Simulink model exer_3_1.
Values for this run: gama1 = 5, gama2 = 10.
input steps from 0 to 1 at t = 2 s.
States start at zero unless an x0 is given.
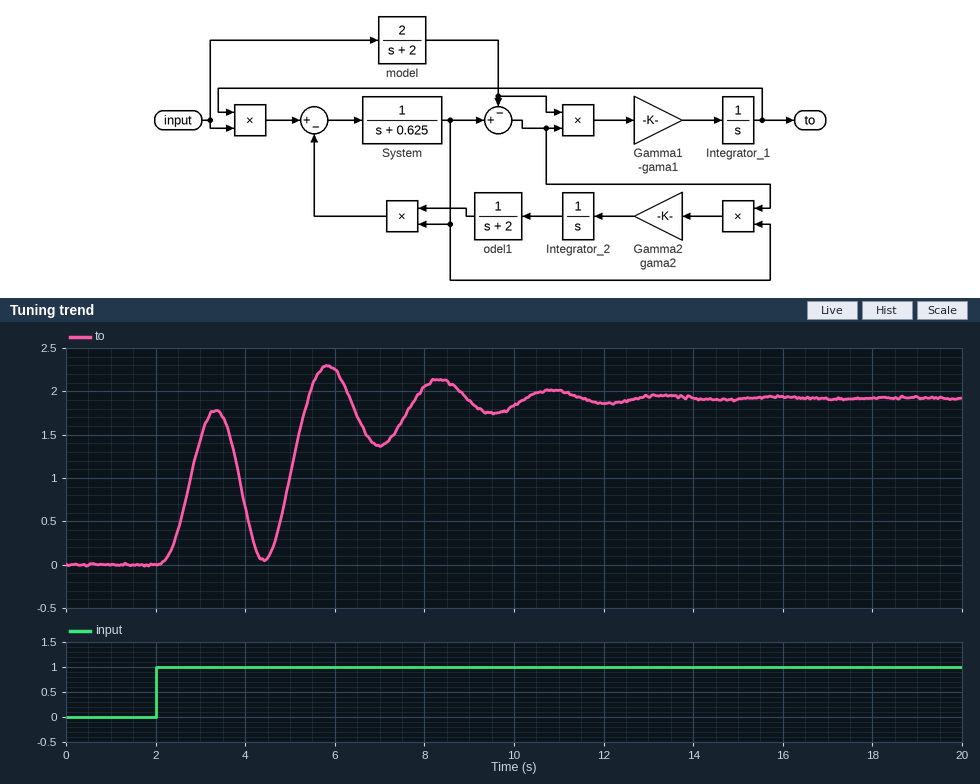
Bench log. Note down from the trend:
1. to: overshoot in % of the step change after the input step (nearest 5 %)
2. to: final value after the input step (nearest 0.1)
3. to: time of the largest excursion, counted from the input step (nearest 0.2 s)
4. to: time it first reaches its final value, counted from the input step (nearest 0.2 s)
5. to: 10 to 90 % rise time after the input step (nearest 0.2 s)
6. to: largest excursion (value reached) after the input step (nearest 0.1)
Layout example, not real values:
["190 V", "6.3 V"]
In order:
["20 %", "1.9", "3.8 s", "3.4 s", "0.8 s", "2.3"]
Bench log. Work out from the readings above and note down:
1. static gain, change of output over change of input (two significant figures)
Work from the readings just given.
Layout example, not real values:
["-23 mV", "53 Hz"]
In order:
["1.9"]
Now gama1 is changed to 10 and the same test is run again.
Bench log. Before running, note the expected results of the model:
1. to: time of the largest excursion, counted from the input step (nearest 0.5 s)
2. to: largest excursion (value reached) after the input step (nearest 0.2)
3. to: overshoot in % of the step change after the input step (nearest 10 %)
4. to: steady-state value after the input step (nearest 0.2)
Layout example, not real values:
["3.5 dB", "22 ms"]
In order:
["3.0 s", "2.4", "40 %", "1.8"]
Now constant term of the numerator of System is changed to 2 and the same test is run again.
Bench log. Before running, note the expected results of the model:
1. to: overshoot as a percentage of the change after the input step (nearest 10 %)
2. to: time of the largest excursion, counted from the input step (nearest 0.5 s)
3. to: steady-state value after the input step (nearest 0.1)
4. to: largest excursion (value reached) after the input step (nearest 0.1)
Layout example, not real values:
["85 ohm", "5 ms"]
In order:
["20 %", "3.0 s", "1.3", "1.5"]
